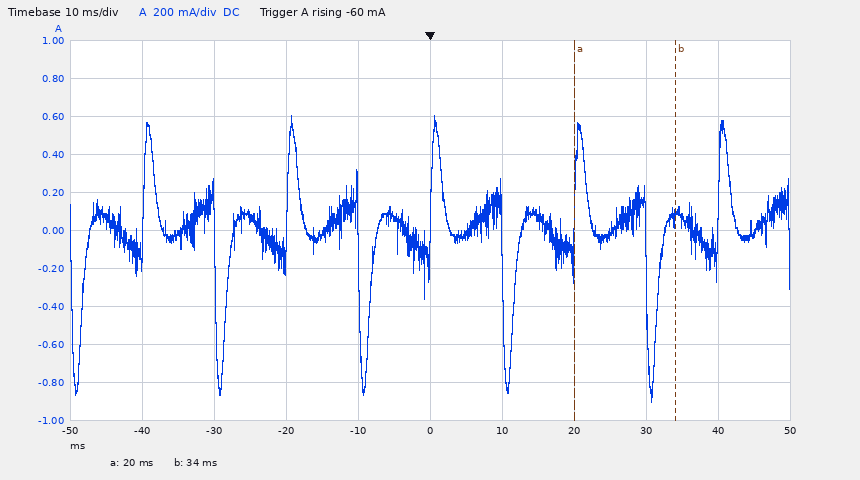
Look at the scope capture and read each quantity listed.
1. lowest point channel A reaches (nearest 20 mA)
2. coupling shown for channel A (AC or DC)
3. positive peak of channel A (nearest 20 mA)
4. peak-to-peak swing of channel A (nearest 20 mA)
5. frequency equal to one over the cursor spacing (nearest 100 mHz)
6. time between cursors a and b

-900 mA
DC
600 mA
1.50 A
71.4 Hz
14 ms
